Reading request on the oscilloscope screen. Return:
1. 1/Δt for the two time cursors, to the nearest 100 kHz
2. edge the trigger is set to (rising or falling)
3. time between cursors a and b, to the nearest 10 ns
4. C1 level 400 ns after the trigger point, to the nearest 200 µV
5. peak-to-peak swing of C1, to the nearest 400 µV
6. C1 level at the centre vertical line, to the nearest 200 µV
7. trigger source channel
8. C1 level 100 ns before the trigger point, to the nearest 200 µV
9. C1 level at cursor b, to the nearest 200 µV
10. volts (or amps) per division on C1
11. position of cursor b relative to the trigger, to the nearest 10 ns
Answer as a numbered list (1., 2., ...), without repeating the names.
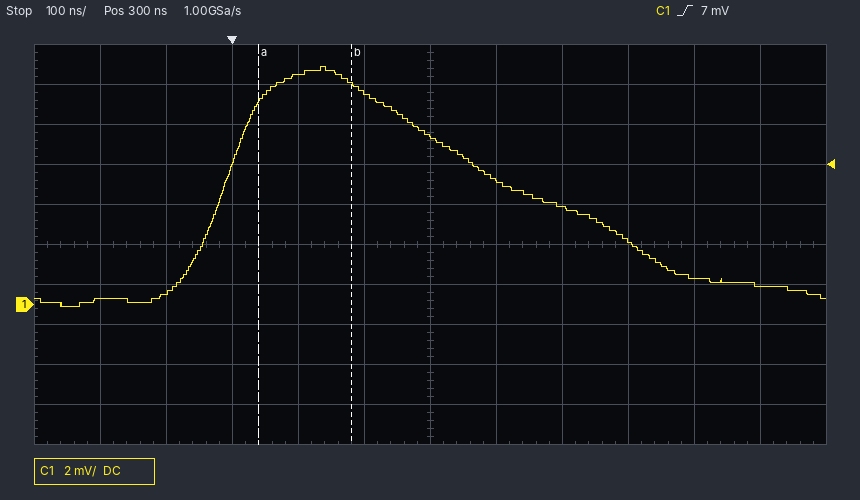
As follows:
1. 7.1 MHz
2. rising
3. 140 ns
4. 6.2 mV
5. 12.0 mV
6. 8.4 mV
7. C1
8. 600 µV
9. 11.0 mV
10. 2 mV
11. +180 ns
